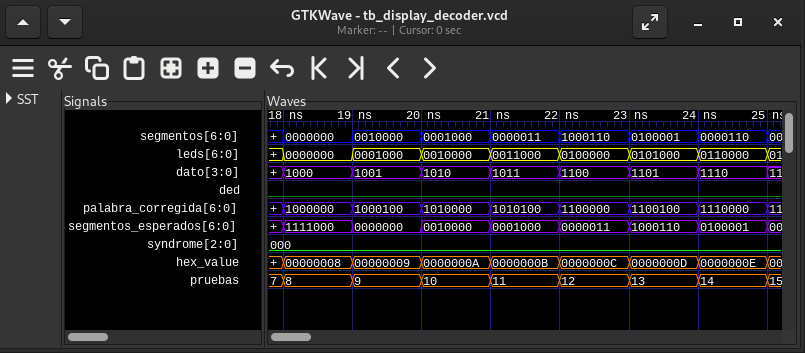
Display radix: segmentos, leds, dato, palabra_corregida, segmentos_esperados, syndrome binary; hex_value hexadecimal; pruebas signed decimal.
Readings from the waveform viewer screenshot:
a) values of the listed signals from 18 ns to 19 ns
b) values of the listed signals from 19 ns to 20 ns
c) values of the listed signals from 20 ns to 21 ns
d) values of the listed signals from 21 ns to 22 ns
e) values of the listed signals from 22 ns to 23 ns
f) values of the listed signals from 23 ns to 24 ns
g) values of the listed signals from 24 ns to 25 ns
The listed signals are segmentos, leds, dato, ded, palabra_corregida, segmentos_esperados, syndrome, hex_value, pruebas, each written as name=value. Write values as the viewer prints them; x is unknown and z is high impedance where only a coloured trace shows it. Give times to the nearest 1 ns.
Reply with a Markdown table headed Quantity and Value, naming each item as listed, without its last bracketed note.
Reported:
| Quantity | Value |
|---|---|
| values of the listed signals from 18 ns to 19 ns | segmentos=0000000, leds=0000000, dato=1000, ded=0, palabra_corregida=1000000, segmentos_esperados=1111000, syndrome=000, hex_value=00000008, pruebas=8 |
| values of the listed signals from 19 ns to 20 ns | segmentos=0010000, leds=0001000, dato=1001, ded=0, palabra_corregida=1000100, segmentos_esperados=0000000, syndrome=000, hex_value=00000009, pruebas=9 |
| values of the listed signals from 20 ns to 21 ns | segmentos=0001000, leds=0010000, dato=1010, ded=0, palabra_corregida=1010000, segmentos_esperados=0010000, syndrome=000, hex_value=0000000A, pruebas=10 |
| values of the listed signals from 21 ns to 22 ns | segmentos=0000011, leds=0011000, dato=1011, ded=0, palabra_corregida=1010100, segmentos_esperados=0001000, syndrome=000, hex_value=0000000B, pruebas=11 |
| values of the listed signals from 22 ns to 23 ns | segmentos=1000110, leds=0100000, dato=1100, ded=0, palabra_corregida=1100000, segmentos_esperados=0000011, syndrome=000, hex_value=0000000C, pruebas=12 |
| values of the listed signals from 23 ns to 24 ns | segmentos=0100001, leds=0101000, dato=1101, ded=0, palabra_corregida=1100100, segmentos_esperados=1000110, syndrome=000, hex_value=0000000D, pruebas=13 |
| values of the listed signals from 24 ns to 25 ns | segmentos=0000110, leds=0110000, dato=1110, ded=0, palabra_corregida=1110000, segmentos_esperados=0100001, syndrome=000, hex_value=0000000E, pruebas=14 |
